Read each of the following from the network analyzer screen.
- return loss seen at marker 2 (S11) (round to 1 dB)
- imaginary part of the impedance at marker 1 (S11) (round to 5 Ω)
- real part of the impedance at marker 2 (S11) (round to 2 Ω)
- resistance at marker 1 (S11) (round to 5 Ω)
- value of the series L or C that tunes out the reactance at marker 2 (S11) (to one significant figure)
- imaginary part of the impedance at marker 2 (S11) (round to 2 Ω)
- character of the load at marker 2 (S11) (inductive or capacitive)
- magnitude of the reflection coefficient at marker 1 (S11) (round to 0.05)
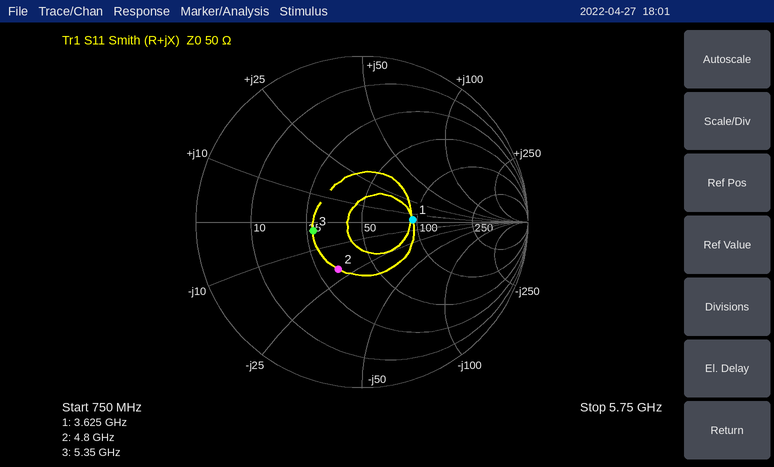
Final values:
10 dB
+5 Ω
32 Ω
95 Ω
700 pH
-20 Ω
capacitive
0.30
